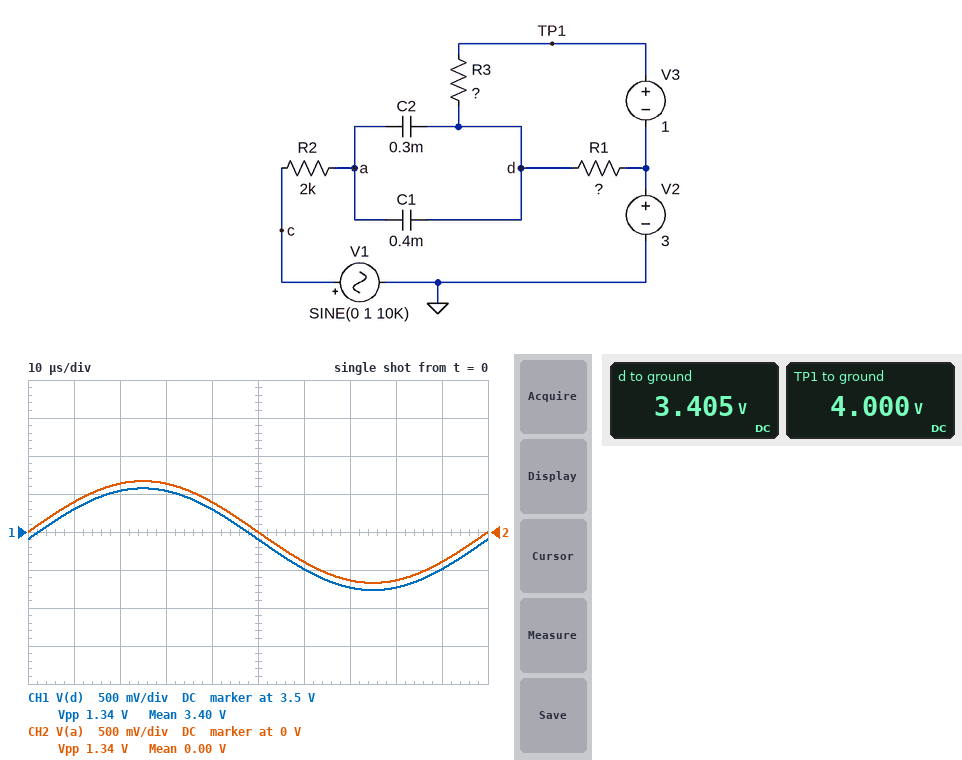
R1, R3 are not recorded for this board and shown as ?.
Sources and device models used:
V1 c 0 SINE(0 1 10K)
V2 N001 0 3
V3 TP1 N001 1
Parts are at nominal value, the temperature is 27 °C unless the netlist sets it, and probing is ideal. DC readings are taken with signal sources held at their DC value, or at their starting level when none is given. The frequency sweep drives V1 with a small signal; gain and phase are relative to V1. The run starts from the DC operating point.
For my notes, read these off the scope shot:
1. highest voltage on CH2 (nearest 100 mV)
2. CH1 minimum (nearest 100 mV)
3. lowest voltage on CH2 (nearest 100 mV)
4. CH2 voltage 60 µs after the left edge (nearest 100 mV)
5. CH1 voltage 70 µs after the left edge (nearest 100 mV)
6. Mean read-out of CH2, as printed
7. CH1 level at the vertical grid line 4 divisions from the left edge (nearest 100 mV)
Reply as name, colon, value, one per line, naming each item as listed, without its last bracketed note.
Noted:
highest voltage on CH2: 700 mV
CH1 minimum: 2.7 V
lowest voltage on CH2: -700 mV
CH2 voltage 60 µs after the left edge: -400 mV
CH1 voltage 70 µs after the left edge: 2.8 V
Mean read-out of CH2, as printed: 0.00 V
CH1 level at the vertical grid line 4 divisions from the left edge: 3.8 V
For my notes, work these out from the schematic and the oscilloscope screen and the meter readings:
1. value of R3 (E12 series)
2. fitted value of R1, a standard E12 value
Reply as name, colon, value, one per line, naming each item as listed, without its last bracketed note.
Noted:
value of R3: 10 kΩ
fitted value of R1, a standard E12 value: 6.8 kΩ
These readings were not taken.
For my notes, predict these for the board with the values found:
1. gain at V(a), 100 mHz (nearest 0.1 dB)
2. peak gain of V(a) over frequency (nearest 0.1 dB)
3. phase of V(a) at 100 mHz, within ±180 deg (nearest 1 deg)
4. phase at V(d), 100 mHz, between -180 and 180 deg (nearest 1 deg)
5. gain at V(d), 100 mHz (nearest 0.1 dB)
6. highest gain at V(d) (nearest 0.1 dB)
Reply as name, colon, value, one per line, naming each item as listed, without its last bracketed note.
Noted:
gain at V(a), 100 mHz: -2.9 dB
peak gain of V(a) over frequency: 0 dB
phase of V(a) at 100 mHz, within ±180 deg: -9 deg
phase at V(d), 100 mHz, between -180 and 180 deg: 21 deg
gain at V(d), 100 mHz: -4.1 dB
highest gain at V(d): -3.5 dB
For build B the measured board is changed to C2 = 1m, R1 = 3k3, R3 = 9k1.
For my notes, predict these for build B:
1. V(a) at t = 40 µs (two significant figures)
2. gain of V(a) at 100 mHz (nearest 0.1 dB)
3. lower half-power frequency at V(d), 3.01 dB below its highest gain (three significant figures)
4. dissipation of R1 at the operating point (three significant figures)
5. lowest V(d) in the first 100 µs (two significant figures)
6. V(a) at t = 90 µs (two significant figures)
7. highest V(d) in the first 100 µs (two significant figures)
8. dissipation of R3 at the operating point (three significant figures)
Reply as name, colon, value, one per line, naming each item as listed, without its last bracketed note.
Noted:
V(a) at t = 40 µs: 320 mV
gain of V(a) at 100 mHz: -4.6 dB
lower half-power frequency at V(d), 3.01 dB below its highest gain: 25.7 mHz
dissipation of R1 at the operating point: 21.5 µW
lowest V(d) in the first 100 µs: 2.7 V
V(a) at t = 90 µs: -320 mV
highest V(d) in the first 100 µs: 3.8 V
dissipation of R3 at the operating point: 59.2 µW
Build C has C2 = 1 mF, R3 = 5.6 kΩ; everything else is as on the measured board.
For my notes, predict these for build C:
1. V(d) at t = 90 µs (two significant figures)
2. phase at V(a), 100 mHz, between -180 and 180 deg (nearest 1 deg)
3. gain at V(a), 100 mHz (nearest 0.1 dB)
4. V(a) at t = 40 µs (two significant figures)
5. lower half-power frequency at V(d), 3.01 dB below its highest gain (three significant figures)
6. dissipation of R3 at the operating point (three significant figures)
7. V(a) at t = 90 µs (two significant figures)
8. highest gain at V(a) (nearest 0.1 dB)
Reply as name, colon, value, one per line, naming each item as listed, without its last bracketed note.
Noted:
V(d) at t = 90 µs: 3.2 V
phase at V(a), 100 mHz, between -180 and 180 deg: -8 deg
gain at V(a), 100 mHz: -4.0 dB
V(a) at t = 40 µs: 360 mV
lower half-power frequency at V(d), 3.01 dB below its highest gain: 22.4 mHz
dissipation of R3 at the operating point: 36.4 µW
V(a) at t = 90 µs: -360 mV
highest gain at V(a): 0 dB
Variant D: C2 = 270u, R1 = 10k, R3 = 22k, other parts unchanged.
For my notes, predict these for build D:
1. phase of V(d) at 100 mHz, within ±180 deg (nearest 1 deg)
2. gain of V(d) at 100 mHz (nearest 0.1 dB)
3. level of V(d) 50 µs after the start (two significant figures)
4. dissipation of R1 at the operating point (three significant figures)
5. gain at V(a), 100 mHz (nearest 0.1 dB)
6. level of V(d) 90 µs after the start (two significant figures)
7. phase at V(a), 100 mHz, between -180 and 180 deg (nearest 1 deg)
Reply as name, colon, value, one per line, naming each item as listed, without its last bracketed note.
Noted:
phase of V(d) at 100 mHz, within ±180 deg: 15 deg
gain of V(d) at 100 mHz: -2.5 dB
level of V(d) 50 µs after the start: 3.3 V
dissipation of R1 at the operating point: 9.77 µW
gain at V(a), 100 mHz: -2.0 dB
level of V(d) 90 µs after the start: 2.9 V
phase at V(a), 100 mHz, between -180 and 180 deg: -4 deg
